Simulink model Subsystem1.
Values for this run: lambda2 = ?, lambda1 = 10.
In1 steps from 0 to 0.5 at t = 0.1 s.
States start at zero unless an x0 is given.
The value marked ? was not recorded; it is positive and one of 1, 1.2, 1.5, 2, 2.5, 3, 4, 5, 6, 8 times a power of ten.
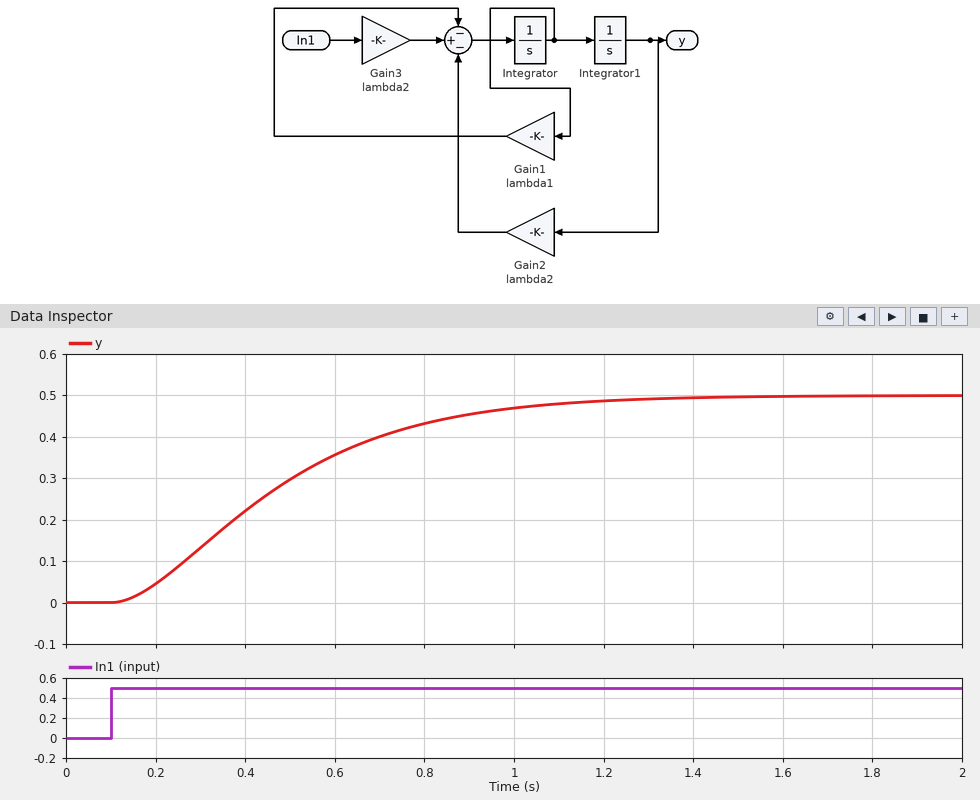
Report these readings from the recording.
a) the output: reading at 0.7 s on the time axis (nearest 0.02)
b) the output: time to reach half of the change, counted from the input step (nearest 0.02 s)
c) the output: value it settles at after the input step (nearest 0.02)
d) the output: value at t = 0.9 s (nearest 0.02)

0.40
0.34 s
0.50
0.46
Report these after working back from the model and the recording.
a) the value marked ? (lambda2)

25
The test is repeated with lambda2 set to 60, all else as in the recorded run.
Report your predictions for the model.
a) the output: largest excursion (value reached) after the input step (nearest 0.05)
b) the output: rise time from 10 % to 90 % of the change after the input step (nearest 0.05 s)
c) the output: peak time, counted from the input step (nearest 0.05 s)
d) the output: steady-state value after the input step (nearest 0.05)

0.55
0.25 s
0.55 s
0.50
